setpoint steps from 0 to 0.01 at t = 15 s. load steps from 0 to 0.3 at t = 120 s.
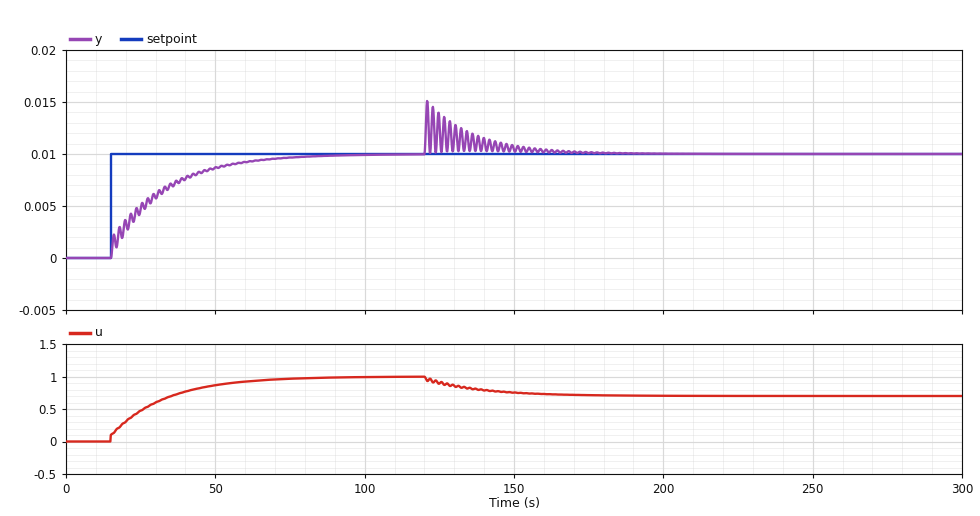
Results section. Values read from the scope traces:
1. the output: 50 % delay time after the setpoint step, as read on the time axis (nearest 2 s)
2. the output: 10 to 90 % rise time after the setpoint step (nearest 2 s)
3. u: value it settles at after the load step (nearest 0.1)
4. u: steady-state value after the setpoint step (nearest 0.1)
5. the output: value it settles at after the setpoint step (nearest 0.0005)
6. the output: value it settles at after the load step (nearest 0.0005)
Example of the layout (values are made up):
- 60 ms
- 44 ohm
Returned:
- 26 s
- 40 s
- 0.7
- 1.0
- 0.0100
- 0.0100
